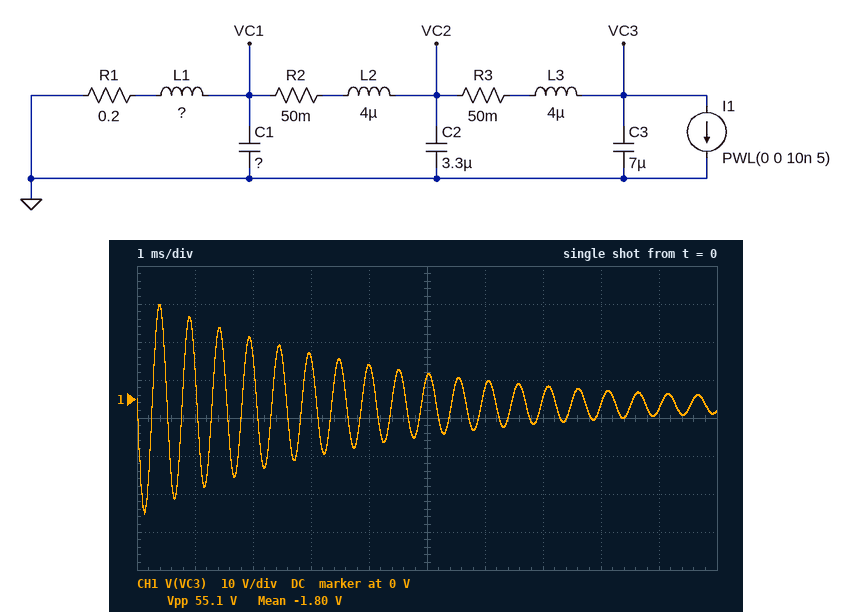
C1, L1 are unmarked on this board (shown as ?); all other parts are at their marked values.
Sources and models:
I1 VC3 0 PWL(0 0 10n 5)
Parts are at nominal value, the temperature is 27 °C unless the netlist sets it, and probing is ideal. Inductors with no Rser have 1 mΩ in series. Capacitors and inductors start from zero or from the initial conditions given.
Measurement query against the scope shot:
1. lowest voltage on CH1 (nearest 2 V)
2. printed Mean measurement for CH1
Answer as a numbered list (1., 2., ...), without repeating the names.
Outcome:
1. -30 V
2. -1.80 V
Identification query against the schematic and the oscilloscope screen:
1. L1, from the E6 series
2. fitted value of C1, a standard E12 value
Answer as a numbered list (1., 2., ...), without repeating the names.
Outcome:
1. 470 µH
2. 3.9 µF
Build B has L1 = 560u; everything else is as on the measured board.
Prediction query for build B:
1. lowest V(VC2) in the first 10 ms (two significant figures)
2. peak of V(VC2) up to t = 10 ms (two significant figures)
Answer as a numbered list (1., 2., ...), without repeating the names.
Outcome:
1. -32 V
2. 28 V
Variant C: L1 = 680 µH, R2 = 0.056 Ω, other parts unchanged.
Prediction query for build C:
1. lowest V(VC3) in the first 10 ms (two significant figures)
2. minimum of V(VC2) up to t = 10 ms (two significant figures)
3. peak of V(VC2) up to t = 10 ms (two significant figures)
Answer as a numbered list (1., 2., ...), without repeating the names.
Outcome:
1. -36 V
2. -35 V
3. 31 V
